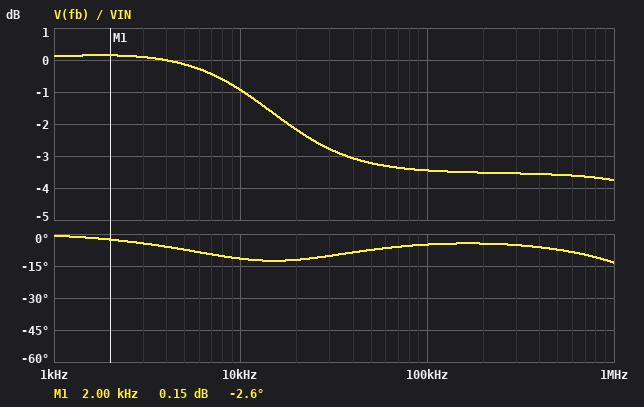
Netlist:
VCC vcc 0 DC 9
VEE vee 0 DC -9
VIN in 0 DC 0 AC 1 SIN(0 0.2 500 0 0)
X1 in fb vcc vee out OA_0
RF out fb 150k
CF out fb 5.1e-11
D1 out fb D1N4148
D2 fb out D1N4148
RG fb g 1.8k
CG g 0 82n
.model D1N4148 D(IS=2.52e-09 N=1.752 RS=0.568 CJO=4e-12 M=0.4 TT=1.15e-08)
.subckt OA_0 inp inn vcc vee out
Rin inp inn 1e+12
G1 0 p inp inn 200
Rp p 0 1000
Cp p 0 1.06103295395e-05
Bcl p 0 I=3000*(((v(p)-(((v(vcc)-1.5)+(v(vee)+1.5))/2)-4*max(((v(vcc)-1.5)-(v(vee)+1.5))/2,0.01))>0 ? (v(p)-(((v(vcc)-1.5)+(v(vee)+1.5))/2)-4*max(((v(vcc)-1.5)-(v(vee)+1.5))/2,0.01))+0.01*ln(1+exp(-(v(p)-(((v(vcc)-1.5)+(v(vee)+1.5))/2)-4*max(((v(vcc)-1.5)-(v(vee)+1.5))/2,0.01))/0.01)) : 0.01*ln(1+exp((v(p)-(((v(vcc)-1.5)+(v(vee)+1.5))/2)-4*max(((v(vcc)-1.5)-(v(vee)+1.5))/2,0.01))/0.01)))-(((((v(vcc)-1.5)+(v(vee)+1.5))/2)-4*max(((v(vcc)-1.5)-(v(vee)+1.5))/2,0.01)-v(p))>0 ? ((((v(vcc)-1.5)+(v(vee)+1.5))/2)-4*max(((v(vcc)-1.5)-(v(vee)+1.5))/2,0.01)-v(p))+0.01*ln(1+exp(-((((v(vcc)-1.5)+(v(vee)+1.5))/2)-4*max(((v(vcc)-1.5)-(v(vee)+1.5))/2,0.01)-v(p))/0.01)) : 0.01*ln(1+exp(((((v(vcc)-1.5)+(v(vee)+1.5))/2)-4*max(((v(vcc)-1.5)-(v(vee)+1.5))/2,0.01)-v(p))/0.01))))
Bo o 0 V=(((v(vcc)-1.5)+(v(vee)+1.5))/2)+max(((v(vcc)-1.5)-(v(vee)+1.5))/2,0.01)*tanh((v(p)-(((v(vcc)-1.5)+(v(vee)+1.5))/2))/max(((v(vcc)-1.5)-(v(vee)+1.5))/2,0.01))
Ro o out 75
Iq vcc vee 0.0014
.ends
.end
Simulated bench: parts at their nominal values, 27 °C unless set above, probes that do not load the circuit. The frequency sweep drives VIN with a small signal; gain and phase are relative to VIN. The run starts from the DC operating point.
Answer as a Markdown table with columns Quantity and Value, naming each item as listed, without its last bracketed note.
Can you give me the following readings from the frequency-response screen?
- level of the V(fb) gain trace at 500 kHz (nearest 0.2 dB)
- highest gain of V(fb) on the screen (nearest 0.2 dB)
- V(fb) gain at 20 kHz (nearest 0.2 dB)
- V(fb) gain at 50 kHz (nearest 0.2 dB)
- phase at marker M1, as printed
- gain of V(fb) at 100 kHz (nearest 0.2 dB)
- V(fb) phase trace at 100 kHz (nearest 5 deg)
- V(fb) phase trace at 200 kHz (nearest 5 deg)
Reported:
| Quantity | Value |
|---|---|
| level of the V(fb) gain trace at 500 kHz | -3.6 dB |
| highest gain of V(fb) on the screen | 0.2 dB |
| V(fb) gain at 20 kHz | -2.2 dB |
| V(fb) gain at 50 kHz | -3.2 dB |
| phase at marker M1, as printed | -2.6 deg |
| gain of V(fb) at 100 kHz | -3.4 dB |
| V(fb) phase trace at 100 kHz | -5 deg |
| V(fb) phase trace at 200 kHz | -5 deg |
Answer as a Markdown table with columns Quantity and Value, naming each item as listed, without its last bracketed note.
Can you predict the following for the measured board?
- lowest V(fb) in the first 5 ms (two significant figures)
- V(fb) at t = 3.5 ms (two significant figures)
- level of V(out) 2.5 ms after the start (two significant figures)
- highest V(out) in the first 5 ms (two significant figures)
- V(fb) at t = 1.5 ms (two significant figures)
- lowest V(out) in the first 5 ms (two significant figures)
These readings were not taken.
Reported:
| Quantity | Value |
|---|---|
| lowest V(fb) in the first 5 ms | -200 mV |
| V(fb) at t = 3.5 ms | -200 mV |
| level of V(out) 2.5 ms after the start | 600 mV |
| highest V(out) in the first 5 ms | 610 mV |
| V(fb) at t = 1.5 ms | -200 mV |
| lowest V(out) in the first 5 ms | -610 mV |
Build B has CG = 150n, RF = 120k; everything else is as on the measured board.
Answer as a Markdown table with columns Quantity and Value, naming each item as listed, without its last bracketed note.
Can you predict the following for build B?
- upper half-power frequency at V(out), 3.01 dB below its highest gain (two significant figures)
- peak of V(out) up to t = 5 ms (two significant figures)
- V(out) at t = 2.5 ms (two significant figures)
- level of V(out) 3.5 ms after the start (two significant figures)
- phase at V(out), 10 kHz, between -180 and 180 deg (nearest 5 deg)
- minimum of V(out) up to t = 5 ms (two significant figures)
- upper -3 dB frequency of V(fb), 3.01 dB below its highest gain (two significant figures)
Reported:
| Quantity | Value |
|---|---|
| upper half-power frequency at V(out), 3.01 dB below its highest gain | 16 kHz |
| peak of V(out) up to t = 5 ms | 650 mV |
| V(out) at t = 2.5 ms | 640 mV |
| level of V(out) 3.5 ms after the start | -640 mV |
| phase at V(out), 10 kHz, between -180 and 180 deg | -30 deg |
| minimum of V(out) up to t = 5 ms | -650 mV |
| upper -3 dB frequency of V(fb), 3.01 dB below its highest gain | 42 kHz |
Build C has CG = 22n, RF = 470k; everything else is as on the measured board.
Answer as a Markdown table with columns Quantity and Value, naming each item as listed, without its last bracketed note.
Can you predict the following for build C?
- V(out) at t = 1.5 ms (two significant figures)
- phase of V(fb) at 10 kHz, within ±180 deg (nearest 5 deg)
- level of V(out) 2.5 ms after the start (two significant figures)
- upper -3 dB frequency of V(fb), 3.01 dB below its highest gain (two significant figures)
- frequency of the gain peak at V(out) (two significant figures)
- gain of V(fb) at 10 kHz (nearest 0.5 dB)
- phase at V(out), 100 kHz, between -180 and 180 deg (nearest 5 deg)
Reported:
| Quantity | Value |
|---|---|
| V(out) at t = 1.5 ms | -480 mV |
| phase of V(fb) at 10 kHz, within ±180 deg | -15 deg |
| level of V(out) 2.5 ms after the start | 480 mV |
| upper -3 dB frequency of V(fb), 3.01 dB below its highest gain | 12 kHz |
| frequency of the gain peak at V(out) | 4.0 kHz |
| gain of V(fb) at 10 kHz | -2.0 dB |
| phase at V(out), 100 kHz, between -180 and 180 deg | -85 deg |
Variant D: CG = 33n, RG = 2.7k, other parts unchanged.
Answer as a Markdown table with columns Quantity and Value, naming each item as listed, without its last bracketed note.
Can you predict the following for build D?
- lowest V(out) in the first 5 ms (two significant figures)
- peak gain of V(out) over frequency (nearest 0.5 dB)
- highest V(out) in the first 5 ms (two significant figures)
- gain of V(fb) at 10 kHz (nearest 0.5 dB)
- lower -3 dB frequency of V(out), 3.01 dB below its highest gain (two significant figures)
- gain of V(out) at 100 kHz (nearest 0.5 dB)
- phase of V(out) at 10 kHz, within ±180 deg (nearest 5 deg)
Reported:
| Quantity | Value |
|---|---|
| lowest V(out) in the first 5 ms | -560 mV |
| peak gain of V(out) over frequency | 34.0 dB |
| highest V(out) in the first 5 ms | 560 mV |
| gain of V(fb) at 10 kHz | -0.5 dB |
| lower -3 dB frequency of V(out), 3.01 dB below its highest gain | 1.5 kHz |
| gain of V(out) at 100 kHz | 17.5 dB |
| phase of V(out) at 10 kHz, within ±180 deg | -25 deg |
